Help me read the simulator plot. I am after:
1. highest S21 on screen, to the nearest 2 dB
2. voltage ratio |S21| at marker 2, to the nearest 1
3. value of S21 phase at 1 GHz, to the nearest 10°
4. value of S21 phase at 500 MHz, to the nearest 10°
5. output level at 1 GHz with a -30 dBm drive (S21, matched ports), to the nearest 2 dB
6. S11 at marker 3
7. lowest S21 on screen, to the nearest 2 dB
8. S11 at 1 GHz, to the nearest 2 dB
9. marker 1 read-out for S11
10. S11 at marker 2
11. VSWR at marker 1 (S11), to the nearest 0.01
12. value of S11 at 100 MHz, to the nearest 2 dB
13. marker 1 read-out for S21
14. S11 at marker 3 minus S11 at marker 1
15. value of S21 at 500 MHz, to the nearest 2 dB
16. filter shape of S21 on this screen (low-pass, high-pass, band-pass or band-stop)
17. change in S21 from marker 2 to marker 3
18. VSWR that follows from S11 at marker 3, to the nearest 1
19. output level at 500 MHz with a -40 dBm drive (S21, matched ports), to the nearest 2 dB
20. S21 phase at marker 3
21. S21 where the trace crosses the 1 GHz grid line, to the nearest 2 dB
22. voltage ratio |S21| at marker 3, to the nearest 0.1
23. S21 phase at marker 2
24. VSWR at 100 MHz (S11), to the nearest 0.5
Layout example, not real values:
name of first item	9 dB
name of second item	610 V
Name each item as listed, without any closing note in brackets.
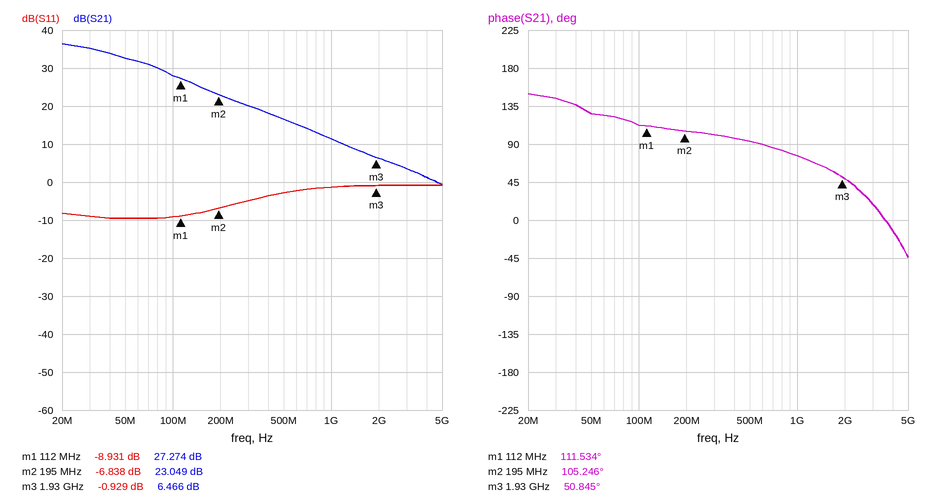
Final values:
highest S21 on screen, to the nearest 2 dB	36 dB
voltage ratio |S21| at marker 2, to the nearest 1	14
value of S21 phase at 1 GHz, to the nearest 10°	80°
value of S21 phase at 500 MHz, to the nearest 10°	90°
output level at 1 GHz with a -30 dBm drive (S21, matched ports), to the nearest 2 dB	-18 dBm
S11 at marker 3	-0.929 dB
lowest S21 on screen, to the nearest 2 dB	0 dB
S11 at 1 GHz, to the nearest 2 dB	-2 dB
marker 1 read-out for S11	-8.931 dB
S11 at marker 2	-6.838 dB
VSWR at marker 1 (S11), to the nearest 0.01	2.11
value of S11 at 100 MHz, to the nearest 2 dB	-10 dB
marker 1 read-out for S21	27.274 dB
S11 at marker 3 minus S11 at marker 1	8.002 dB
value of S21 at 500 MHz, to the nearest 2 dB	16 dB
filter shape of S21 on this screen	low-pass
change in S21 from marker 2 to marker 3	-16.583 dB
VSWR that follows from S11 at marker 3, to the nearest 1	19
output level at 500 MHz with a -40 dBm drive (S21, matched ports), to the nearest 2 dB	-24 dBm
S21 phase at marker 3	50.845°
S21 where the trace crosses the 1 GHz grid line, to the nearest 2 dB	12 dB
voltage ratio |S21| at marker 3, to the nearest 0.1	2.1
S21 phase at marker 2	105.246°
VSWR at 100 MHz (S11), to the nearest 0.5	2.0
